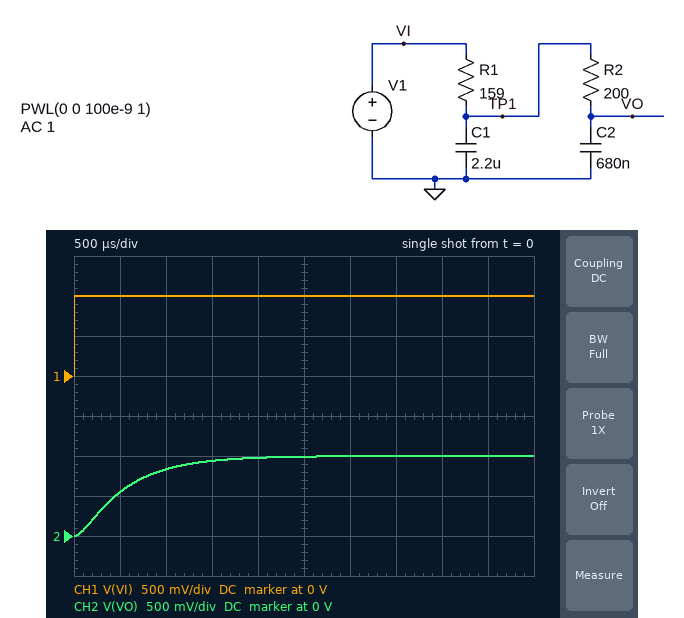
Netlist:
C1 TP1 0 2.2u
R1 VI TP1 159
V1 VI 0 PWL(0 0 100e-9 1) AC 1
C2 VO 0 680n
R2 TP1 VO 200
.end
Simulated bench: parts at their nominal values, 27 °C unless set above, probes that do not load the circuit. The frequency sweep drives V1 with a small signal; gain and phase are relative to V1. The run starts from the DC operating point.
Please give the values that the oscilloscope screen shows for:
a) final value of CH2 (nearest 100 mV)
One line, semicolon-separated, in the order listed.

1.0 V
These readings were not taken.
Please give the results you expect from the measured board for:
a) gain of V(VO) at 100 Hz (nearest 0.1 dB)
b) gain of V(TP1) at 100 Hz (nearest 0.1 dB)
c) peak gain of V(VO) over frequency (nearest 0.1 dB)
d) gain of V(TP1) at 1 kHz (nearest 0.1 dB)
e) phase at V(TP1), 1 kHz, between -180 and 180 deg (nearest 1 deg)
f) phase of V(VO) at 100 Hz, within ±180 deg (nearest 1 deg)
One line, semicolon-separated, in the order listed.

-0.4 dB; -0.4 dB; 0 dB; -9.3 dB; -63 deg; -21 deg
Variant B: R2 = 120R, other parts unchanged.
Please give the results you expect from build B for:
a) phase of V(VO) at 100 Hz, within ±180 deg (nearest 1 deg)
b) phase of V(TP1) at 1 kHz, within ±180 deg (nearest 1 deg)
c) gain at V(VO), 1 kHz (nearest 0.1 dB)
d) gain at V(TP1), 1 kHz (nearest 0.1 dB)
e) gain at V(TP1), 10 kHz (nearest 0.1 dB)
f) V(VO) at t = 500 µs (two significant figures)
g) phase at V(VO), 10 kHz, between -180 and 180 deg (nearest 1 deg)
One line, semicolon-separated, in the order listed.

-19 deg; -65 deg; -10.6 dB; -9.6 dB; -27.0 dB; 600 mV; -163 deg
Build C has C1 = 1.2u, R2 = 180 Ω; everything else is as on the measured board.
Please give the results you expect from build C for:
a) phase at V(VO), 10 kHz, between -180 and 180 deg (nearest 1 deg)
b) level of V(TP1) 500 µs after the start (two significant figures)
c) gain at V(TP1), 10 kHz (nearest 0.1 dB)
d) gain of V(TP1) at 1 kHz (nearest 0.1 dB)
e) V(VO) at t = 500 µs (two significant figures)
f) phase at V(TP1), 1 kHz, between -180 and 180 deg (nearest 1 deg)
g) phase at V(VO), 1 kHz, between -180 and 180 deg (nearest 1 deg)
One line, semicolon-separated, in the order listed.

-164 deg; 800 mV; -21.8 dB; -6.4 dB; 700 mV; -51 deg; -88 deg
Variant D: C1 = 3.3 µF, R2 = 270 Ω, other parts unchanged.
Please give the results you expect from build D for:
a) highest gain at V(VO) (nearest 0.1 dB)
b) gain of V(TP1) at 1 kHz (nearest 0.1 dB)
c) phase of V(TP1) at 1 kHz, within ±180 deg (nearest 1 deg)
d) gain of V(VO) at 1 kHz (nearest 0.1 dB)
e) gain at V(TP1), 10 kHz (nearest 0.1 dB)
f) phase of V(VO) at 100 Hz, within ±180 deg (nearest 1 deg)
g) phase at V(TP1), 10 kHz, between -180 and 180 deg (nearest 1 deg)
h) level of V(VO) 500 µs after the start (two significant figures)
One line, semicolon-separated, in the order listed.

0 dB; -11.7 dB; -70 deg; -15.3 dB; -30.4 dB; -28 deg; -87 deg; 400 mV
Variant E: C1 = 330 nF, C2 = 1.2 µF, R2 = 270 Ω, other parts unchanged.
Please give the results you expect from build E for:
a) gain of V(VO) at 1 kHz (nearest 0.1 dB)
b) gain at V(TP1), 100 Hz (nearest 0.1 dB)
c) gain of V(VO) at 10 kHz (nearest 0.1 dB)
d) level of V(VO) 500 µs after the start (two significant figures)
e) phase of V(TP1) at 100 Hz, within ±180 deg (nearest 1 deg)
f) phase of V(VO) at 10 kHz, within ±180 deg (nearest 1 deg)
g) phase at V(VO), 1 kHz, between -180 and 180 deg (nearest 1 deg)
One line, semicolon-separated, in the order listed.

-11.1 dB; -0.3 dB; -37.5 dB; 580 mV; -8 deg; -152 deg; -85 deg
